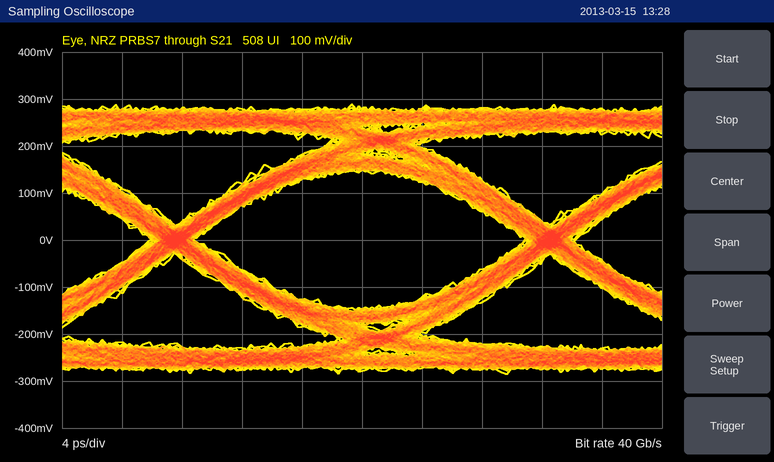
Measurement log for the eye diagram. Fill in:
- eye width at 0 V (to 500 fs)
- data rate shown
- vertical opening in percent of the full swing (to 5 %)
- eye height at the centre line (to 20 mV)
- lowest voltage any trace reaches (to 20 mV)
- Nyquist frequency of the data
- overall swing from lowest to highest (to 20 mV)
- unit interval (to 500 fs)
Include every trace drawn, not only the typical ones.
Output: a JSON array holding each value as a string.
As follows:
["22.0 ps", "40 Gb/s", "50 %", "300 mV", "-280 mV", "20 GHz", "580 mV", "25.0 ps"]
